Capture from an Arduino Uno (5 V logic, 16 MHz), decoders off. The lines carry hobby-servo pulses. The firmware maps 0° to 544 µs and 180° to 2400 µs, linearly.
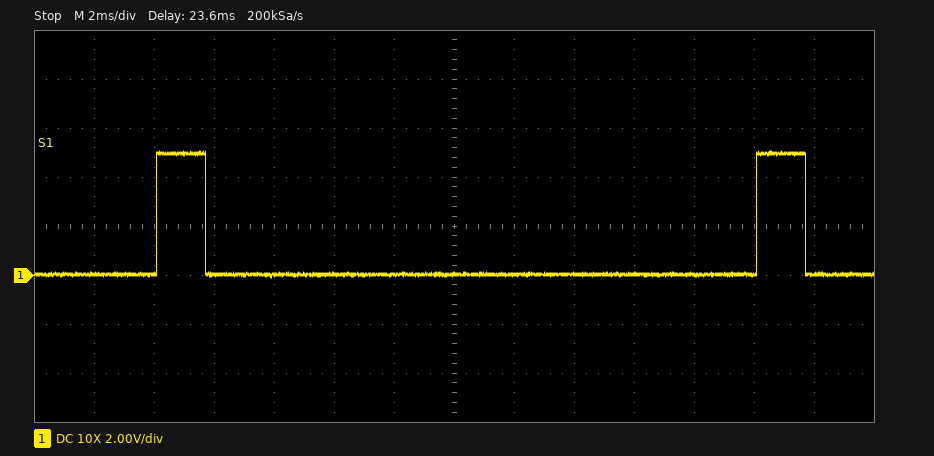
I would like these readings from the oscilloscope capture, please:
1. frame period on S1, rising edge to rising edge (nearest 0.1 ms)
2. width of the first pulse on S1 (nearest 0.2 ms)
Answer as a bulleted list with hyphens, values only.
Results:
- 20.0 ms
- 1.6 ms
